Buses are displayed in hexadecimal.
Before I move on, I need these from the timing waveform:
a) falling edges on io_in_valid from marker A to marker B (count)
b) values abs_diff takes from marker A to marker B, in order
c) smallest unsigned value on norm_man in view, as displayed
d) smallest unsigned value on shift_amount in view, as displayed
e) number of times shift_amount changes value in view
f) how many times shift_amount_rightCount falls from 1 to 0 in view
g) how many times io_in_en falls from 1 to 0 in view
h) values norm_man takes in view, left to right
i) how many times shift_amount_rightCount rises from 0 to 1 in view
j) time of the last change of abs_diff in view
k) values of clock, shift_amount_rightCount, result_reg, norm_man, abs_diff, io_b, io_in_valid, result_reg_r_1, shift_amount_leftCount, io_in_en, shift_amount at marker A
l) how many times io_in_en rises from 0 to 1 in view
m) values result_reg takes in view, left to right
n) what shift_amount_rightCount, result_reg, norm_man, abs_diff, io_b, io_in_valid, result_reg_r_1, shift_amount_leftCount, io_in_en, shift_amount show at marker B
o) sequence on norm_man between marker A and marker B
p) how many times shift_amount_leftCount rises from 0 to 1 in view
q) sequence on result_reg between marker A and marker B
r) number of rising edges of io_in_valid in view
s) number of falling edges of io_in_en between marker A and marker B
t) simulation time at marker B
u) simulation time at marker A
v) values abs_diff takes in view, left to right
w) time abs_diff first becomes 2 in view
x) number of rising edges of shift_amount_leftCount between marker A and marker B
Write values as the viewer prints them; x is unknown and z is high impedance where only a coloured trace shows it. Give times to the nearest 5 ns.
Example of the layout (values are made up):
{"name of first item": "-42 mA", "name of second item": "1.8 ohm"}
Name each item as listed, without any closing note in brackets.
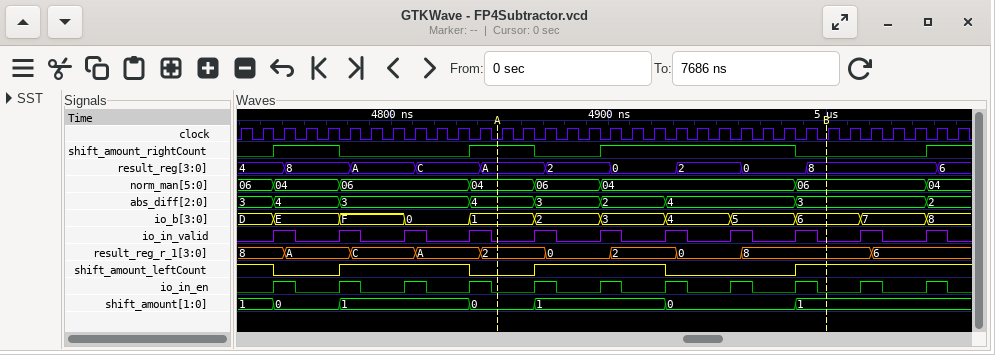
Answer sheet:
{"falling edges on io_in_valid from marker A to marker B": "5", "values abs_diff takes from marker A to marker B, in order": "4, 3, 2, 4, 3", "smallest unsigned value on norm_man in view, as displayed": "04", "smallest unsigned value on shift_amount in view, as displayed": "0", "number of times shift_amount changes value in view": "6", "how many times shift_amount_rightCount falls from 1 to 0 in view": "3", "how many times io_in_en falls from 1 to 0 in view": "11", "values norm_man takes in view, left to right": "06, 04, 06, 04, 06, 04, 06, 04", "how many times shift_amount_rightCount rises from 0 to 1 in view": "4", "time of the last change of abs_diff in view": "5045 ns", "values of clock, shift_amount_rightCount, result_reg, norm_man, abs_diff, io_b, io_in_valid, result_reg_r_1, shift_amount_leftCount, io_in_en, shift_amount at marker A": "clock=0, shift_amount_rightCount=1, result_reg=A, norm_man=04, abs_diff=4, io_b=1, io_in_valid=0, result_reg_r_1=2, shift_amount_leftCount=0, io_in_en=0, shift_amount=0", "how many times io_in_en rises from 0 to 1 in view": "11", "values result_reg takes in view, left to right": "4, 8, A, C, A, 2, 0, 2, 0, 8, 6", "what shift_amount_rightCount, result_reg, norm_man, abs_diff, io_b, io_in_valid, result_reg_r_1, shift_amount_leftCount, io_in_en, shift_amount show at marker B": "shift_amount_rightCount=0, result_reg=8, norm_man=06, abs_diff=3, io_b=6, io_in_valid=0, result_reg_r_1=8, shift_amount_leftCount=1, io_in_en=0, shift_amount=1", "sequence on norm_man between marker A and marker B": "04, 06, 04, 06", "how many times shift_amount_leftCount rises from 0 to 1 in view": "3", "sequence on result_reg between marker A and marker B": "A, 2, 0, 2, 0, 8", "number of rising edges of io_in_valid in view": "11", "number of falling edges of io_in_en between marker A and marker B": "5", "simulation time at marker B": "5000 ns", "simulation time at marker A": "4850 ns", "values abs_diff takes in view, left to right": "3, 4, 3, 4, 3, 2, 4, 3, 2", "time abs_diff first becomes 2 in view": "4895 ns", "number of rising edges of shift_amount_leftCount between marker A and marker B": "2"}
